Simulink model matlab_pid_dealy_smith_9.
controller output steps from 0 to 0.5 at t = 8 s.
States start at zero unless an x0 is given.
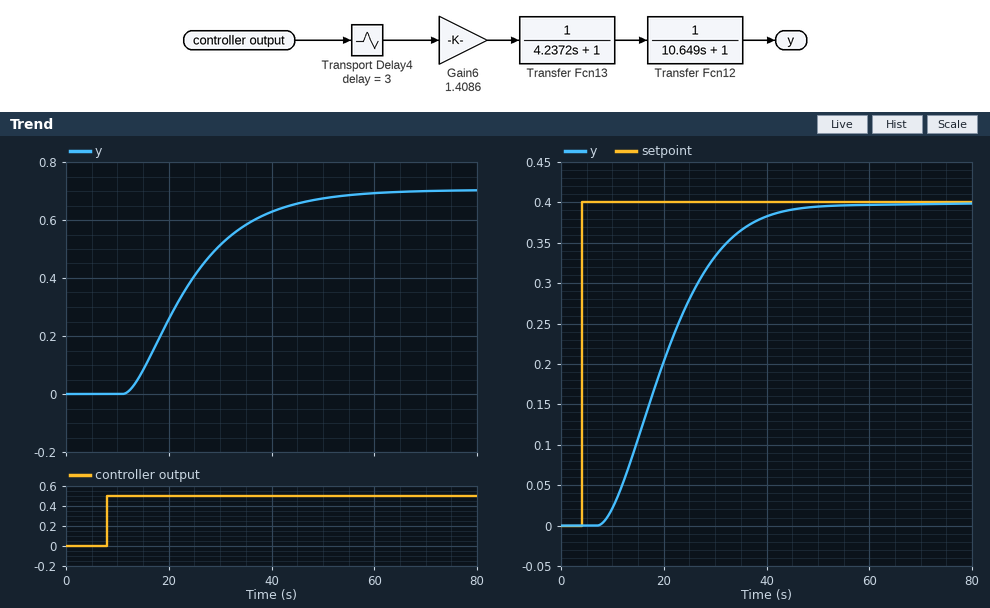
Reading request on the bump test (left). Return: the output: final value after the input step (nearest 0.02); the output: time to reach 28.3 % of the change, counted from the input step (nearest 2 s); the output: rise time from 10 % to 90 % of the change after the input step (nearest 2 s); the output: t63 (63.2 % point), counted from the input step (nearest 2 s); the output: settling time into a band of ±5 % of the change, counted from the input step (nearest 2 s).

0.70
10 s
26 s
18 s
40 s
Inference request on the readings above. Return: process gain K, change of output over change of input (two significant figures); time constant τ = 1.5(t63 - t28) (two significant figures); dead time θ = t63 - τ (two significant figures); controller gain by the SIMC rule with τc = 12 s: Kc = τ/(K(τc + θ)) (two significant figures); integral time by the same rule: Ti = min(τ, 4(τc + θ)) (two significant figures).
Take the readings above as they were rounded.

1.4
12 s
6.0 s
0.48
12 s
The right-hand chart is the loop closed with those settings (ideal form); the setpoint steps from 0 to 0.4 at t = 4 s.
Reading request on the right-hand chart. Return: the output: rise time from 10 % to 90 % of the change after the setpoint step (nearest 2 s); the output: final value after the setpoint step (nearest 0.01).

22 s
0.40
